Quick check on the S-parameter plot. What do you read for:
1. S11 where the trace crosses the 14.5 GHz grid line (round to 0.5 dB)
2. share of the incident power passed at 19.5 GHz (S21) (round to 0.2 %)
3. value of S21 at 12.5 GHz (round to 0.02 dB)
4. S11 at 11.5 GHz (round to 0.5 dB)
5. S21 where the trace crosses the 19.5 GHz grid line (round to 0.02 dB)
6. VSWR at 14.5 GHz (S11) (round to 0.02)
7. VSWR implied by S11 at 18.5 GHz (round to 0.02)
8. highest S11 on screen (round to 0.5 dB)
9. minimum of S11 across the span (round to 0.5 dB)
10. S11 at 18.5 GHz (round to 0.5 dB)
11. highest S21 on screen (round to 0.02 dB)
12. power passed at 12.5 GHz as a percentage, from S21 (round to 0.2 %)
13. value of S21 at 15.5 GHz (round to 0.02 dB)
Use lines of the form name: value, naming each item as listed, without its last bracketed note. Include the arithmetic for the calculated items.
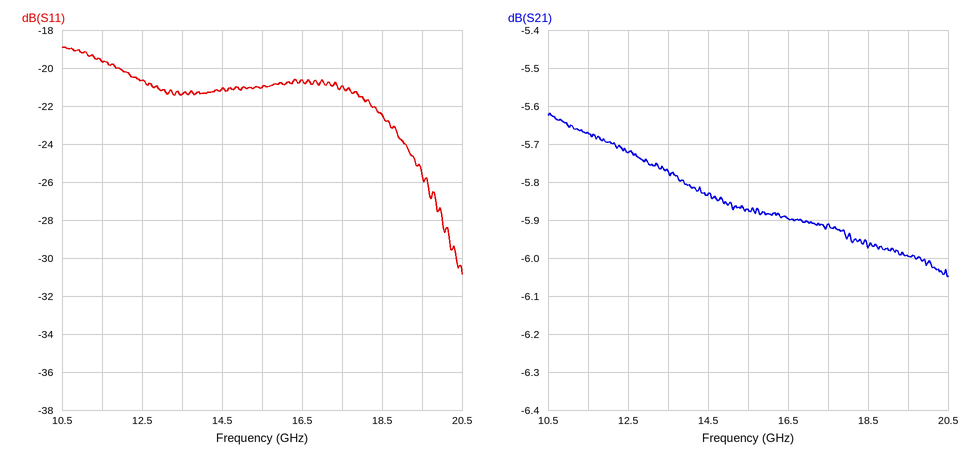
S11 where the trace crosses the 14.5 GHz grid line: -21.0 dB
share of the incident power passed at 19.5 GHz (S21): 10^(-6/10) ≈ 25.1 %, so 25.2 % to the nearest 0.2 %
value of S21 at 12.5 GHz: -5.72 dB
S11 at 11.5 GHz: -19.5 dB
S21 where the trace crosses the 19.5 GHz grid line: -6.00 dB
VSWR at 14.5 GHz (S11): |Γ| = 10^(-21/20) = 0.0891; VSWR = (1 + 0.0891)/(1 − 0.0891) ≈ 1.20
VSWR implied by S11 at 18.5 GHz: |Γ| = 10^(-22.5/20) = 0.0750; VSWR = (1 + 0.0750)/(1 − 0.0750) ≈ 1.16
highest S11 on screen: -19.0 dB
minimum of S11 across the span: -31.0 dB
S11 at 18.5 GHz: -22.5 dB
highest S21 on screen: -5.62 dB
power passed at 12.5 GHz as a percentage, from S21: 10^(-5.72/10) ≈ 26.8 %
value of S21 at 15.5 GHz: -5.88 dB
